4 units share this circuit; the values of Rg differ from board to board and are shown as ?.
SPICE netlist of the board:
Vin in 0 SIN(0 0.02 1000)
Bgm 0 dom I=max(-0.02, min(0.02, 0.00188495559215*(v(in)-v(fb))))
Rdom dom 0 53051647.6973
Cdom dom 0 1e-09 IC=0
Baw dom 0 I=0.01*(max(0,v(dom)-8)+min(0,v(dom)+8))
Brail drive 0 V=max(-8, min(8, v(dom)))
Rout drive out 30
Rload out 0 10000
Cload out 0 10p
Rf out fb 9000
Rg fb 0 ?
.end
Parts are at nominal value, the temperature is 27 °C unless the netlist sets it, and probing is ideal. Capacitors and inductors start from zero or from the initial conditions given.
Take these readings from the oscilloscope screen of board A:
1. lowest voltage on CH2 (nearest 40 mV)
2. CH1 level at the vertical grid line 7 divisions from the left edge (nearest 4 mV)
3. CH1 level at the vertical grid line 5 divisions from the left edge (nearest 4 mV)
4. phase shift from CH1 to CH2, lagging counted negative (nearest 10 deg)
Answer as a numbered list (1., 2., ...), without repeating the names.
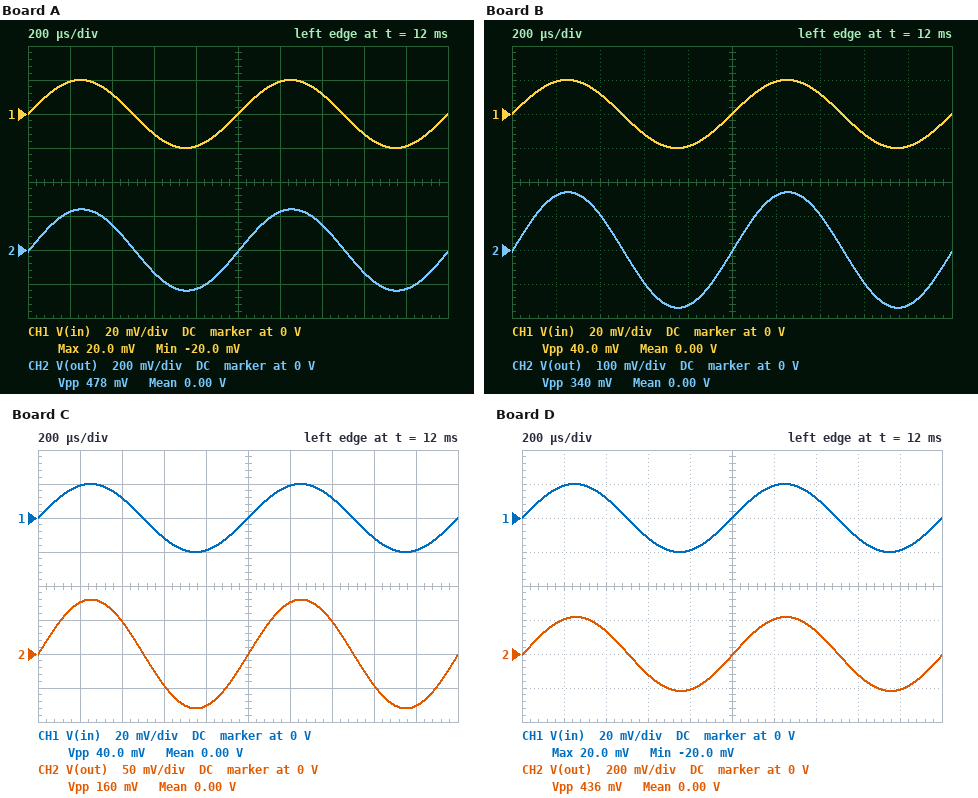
1. -240 mV
2. 12 mV
3. 0 V
4. 0 deg
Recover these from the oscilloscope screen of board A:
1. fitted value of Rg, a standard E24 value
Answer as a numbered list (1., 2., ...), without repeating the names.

1. 820 Ω
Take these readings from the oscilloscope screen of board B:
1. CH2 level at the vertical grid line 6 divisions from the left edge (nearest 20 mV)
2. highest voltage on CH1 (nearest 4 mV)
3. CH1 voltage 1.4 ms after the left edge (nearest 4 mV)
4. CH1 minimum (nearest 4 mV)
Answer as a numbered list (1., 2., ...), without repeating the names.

1. 160 mV
2. 20 mV
3. 12 mV
4. -20 mV
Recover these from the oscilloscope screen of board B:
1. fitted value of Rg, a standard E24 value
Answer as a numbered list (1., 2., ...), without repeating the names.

1. 1.2 kΩ
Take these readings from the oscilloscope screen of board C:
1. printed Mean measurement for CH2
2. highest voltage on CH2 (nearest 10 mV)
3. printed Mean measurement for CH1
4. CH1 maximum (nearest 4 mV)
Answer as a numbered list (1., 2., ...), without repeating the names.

1. 0.00 V
2. 80 mV
3. 0.00 V
4. 20 mV
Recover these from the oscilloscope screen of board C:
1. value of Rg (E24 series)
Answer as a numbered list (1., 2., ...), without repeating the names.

1. 3 kΩ
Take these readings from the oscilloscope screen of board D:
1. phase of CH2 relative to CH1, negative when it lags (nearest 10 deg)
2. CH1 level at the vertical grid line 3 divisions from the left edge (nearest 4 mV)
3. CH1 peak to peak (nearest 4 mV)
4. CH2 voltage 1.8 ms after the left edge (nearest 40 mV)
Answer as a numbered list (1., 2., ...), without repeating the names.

1. 0 deg
2. -12 mV
3. 40 mV
4. -200 mV
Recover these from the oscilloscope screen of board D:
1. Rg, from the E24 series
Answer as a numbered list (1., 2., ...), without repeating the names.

1. 910 Ω
